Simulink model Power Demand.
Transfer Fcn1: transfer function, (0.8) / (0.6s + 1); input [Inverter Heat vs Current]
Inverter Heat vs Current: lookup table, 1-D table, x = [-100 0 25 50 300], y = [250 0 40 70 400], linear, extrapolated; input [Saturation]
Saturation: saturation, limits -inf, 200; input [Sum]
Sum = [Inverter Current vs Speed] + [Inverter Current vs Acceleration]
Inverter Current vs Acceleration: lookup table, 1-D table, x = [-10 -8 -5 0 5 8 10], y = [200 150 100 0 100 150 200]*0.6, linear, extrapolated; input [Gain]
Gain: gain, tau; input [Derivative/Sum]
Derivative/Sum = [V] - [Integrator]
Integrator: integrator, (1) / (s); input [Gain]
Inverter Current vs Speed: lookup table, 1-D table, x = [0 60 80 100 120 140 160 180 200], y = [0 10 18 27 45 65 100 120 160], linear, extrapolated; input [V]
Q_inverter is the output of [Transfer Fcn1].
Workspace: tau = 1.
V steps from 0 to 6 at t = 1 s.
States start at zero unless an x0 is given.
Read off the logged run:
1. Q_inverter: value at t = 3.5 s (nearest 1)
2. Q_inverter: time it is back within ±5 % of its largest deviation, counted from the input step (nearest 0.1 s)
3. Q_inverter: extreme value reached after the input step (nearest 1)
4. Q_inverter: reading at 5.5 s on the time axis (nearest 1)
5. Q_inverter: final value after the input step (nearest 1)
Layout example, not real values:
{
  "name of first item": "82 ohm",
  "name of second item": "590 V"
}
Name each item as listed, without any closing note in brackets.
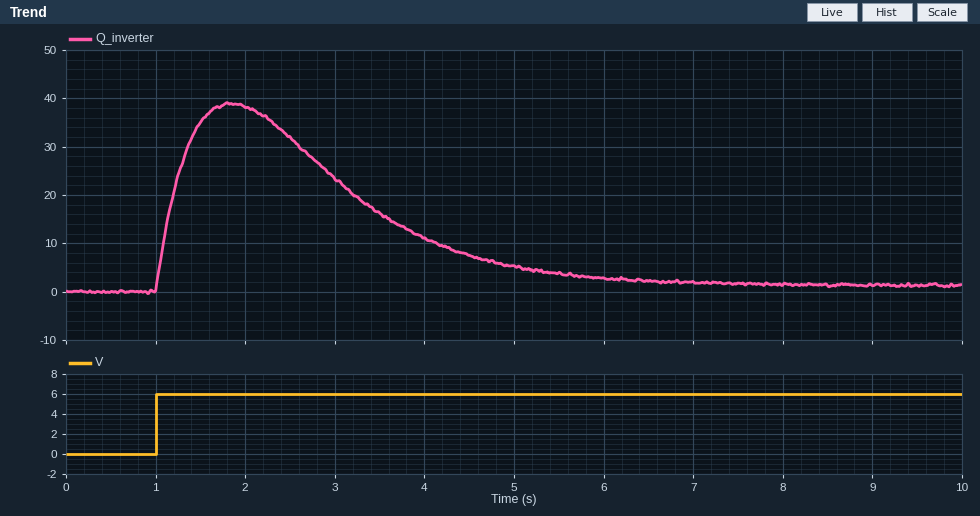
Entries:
{
  "Q_inverter: value at t = 3.5 s": "16",
  "Q_inverter: time it is back within ±5 % of its largest deviation, counted from the input step": "4.7 s",
  "Q_inverter: extreme value reached after the input step": "39",
  "Q_inverter: reading at 5.5 s on the time axis": "4",
  "Q_inverter: final value after the input step": "1"
}
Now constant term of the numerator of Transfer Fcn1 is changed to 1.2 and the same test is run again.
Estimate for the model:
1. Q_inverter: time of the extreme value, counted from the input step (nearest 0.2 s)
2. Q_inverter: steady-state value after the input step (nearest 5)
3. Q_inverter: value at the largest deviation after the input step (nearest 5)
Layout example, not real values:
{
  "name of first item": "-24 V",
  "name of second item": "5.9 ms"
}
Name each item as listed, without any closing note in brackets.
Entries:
{
  "Q_inverter: time of the extreme value, counted from the input step": "0.8 s",
  "Q_inverter: steady-state value after the input step": "0",
  "Q_inverter: value at the largest deviation after the input step": "60"
}
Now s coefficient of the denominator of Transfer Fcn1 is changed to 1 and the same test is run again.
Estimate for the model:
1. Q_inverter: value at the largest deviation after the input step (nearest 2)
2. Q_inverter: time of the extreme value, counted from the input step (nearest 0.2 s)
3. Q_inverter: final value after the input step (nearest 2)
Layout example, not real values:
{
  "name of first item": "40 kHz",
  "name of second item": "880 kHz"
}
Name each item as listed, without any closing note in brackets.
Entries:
{
  "Q_inverter: value at the largest deviation after the input step": "32",
  "Q_inverter: time of the extreme value, counted from the input step": "1.2 s",
  "Q_inverter: final value after the input step": "2"
}
